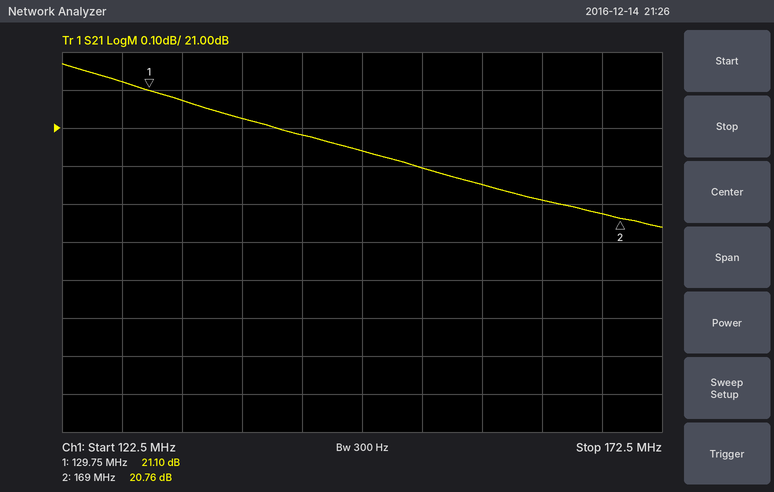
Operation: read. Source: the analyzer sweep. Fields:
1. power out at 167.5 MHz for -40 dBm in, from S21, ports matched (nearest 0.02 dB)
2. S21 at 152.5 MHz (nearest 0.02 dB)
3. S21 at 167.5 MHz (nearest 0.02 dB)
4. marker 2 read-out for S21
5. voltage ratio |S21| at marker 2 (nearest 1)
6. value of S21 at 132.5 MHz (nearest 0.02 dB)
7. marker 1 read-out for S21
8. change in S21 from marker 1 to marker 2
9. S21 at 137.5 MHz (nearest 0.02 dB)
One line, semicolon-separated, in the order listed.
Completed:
-19.22 dBm; 20.90 dB; 20.78 dB; 20.76 dB; 11; 21.08 dB; 21.10 dB; -0.34 dB; 21.02 dB
